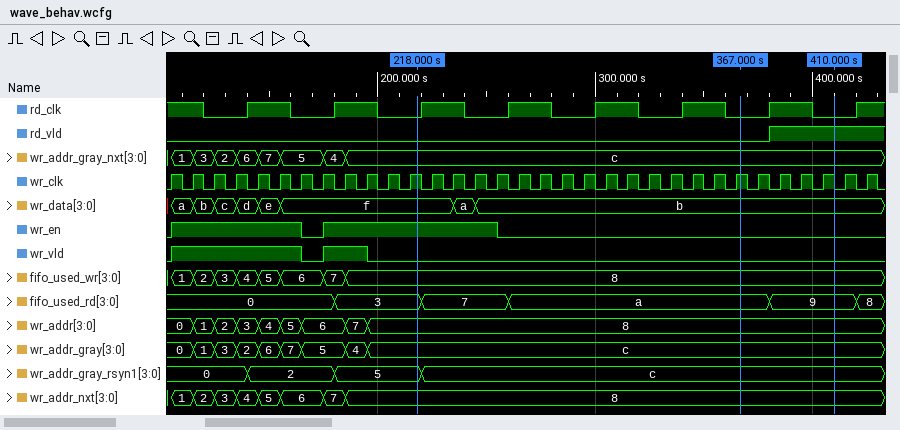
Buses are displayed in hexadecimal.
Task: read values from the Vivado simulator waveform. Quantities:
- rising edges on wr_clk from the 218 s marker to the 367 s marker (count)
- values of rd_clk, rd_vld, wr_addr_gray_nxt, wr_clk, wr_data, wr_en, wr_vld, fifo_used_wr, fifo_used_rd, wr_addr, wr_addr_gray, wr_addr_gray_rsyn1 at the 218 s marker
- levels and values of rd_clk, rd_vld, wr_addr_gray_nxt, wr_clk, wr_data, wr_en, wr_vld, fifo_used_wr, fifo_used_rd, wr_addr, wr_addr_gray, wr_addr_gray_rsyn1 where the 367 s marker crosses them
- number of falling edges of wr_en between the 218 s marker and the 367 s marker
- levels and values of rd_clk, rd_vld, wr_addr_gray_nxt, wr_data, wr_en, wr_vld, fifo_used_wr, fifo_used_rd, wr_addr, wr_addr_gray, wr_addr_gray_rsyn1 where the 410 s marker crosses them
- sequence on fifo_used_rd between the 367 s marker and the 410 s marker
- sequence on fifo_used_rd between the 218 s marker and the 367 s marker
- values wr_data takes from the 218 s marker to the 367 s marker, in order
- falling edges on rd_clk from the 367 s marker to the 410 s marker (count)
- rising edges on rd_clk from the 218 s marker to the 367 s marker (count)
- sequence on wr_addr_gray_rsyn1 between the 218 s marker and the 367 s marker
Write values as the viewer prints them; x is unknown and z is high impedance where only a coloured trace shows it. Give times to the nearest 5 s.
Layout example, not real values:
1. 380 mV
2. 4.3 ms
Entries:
1. 15
2. rd_clk=0, rd_vld=0, wr_addr_gray_nxt=c, wr_clk=1, wr_data=f, wr_en=1, wr_vld=0, fifo_used_wr=8, fifo_used_rd=3, wr_addr=8, wr_addr_gray=c, wr_addr_gray_rsyn1=5
3. rd_clk=0, rd_vld=0, wr_addr_gray_nxt=c, wr_clk=1, wr_data=b, wr_en=0, wr_vld=0, fifo_used_wr=8, fifo_used_rd=a, wr_addr=8, wr_addr_gray=c, wr_addr_gray_rsyn1=c
4. 1
5. rd_clk=0, rd_vld=1, wr_addr_gray_nxt=c, wr_data=b, wr_en=0, wr_vld=0, fifo_used_wr=8, fifo_used_rd=9, wr_addr=8, wr_addr_gray=c, wr_addr_gray_rsyn1=c
6. a, 9
7. 3, 7, a
8. f, a, b
9. 1
10. 4
11. 5, c
